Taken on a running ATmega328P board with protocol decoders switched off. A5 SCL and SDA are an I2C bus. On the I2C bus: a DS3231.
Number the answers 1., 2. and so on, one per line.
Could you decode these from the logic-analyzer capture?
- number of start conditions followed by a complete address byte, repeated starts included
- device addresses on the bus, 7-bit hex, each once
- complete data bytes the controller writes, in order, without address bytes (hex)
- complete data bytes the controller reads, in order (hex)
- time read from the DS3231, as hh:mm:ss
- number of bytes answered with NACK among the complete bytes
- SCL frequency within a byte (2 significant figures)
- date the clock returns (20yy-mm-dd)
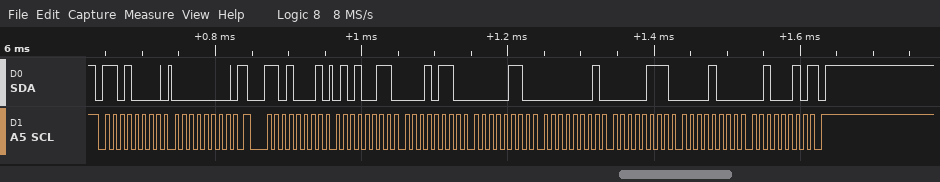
1. 2
2. 0x68
3. 00
4. 53 16 06 01 07 08 22
5. 06:16:53
6. 1
7. 100 kHz
8. 2022-08-07
